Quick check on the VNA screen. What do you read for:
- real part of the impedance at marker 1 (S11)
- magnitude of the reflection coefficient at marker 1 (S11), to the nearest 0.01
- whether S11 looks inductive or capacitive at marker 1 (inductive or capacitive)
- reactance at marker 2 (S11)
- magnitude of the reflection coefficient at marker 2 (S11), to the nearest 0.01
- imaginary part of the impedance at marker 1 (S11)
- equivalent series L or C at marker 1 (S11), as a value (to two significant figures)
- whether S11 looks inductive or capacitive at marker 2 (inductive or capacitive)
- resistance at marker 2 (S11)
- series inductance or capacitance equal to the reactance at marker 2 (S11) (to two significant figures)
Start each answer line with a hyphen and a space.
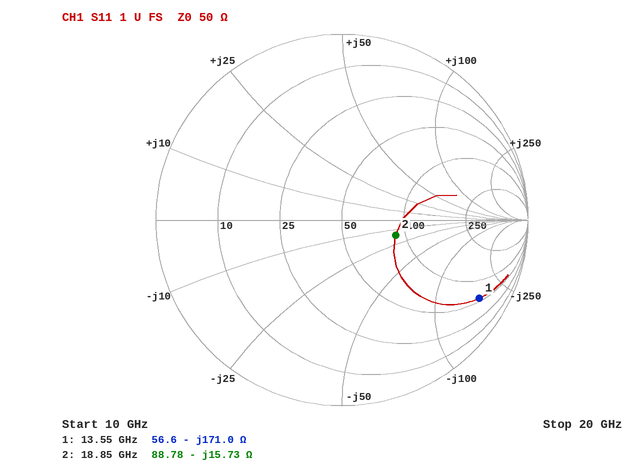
- 56.6 Ω
- 0.85
- capacitive
- -15.73 Ω
- 0.30
- -171.0 Ω
- 69 fF
- capacitive
- 88.78 Ω
- 540 fF
